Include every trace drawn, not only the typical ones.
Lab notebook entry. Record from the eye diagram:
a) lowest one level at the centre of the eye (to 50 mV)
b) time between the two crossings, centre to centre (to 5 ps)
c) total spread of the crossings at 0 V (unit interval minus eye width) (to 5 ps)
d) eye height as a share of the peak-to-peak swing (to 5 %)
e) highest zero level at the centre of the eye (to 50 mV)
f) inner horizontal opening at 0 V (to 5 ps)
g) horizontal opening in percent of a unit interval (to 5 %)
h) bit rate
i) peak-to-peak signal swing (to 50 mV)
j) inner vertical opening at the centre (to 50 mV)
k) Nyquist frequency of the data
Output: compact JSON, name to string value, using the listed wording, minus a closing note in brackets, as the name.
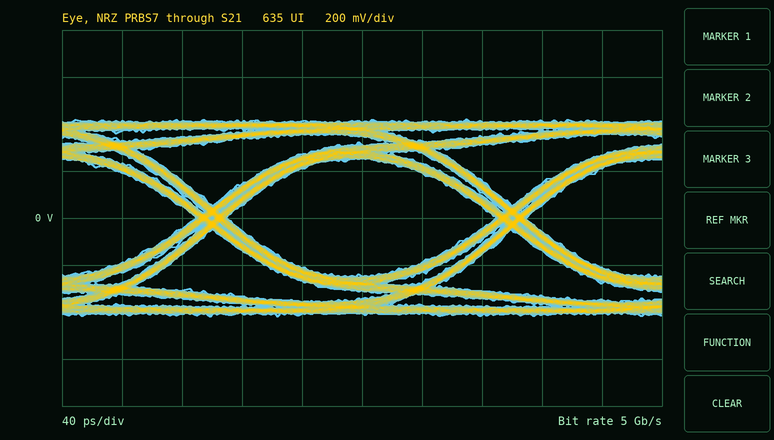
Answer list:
{"lowest one level at the centre of the eye": "250 mV", "time between the two crossings, centre to centre": "200 ps", "total spread of the crossings at 0 V (unit interval minus eye width)": "20 ps", "eye height as a share of the peak-to-peak swing": "60 %", "highest zero level at the centre of the eye": "-250 mV", "inner horizontal opening at 0 V": "180 ps", "horizontal opening in percent of a unit interval": "90 %", "bit rate": "5 Gb/s", "peak-to-peak signal swing": "850 mV", "inner vertical opening at the centre": "500 mV", "Nyquist frequency of the data": "2.5 GHz"}
